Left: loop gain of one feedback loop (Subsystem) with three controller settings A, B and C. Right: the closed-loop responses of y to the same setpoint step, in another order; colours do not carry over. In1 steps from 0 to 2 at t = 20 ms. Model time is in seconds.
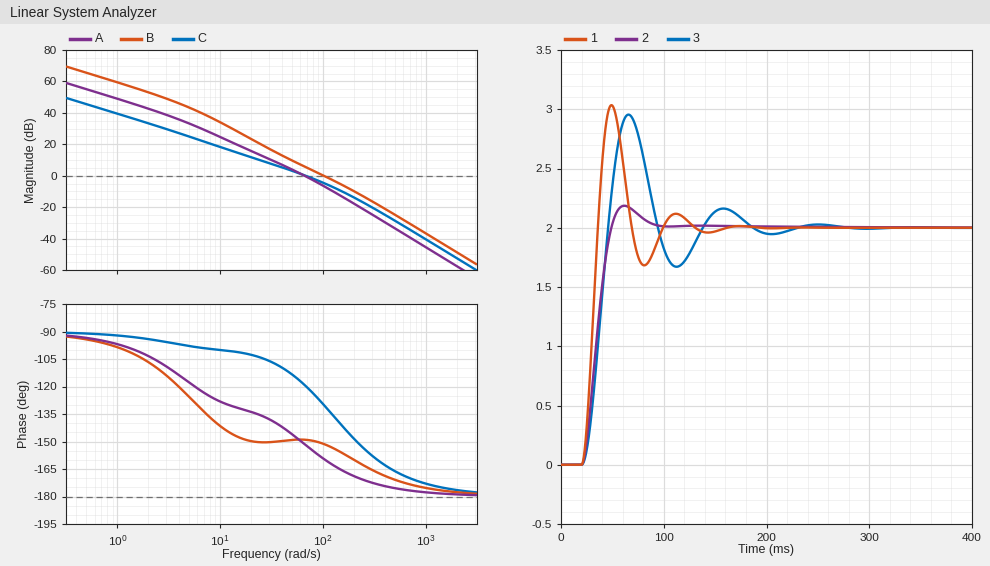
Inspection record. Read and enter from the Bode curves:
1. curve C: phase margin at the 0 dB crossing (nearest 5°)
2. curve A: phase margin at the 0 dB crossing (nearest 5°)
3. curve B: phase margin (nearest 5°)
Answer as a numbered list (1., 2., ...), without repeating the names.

1. 60°
2. 30°
3. 30°
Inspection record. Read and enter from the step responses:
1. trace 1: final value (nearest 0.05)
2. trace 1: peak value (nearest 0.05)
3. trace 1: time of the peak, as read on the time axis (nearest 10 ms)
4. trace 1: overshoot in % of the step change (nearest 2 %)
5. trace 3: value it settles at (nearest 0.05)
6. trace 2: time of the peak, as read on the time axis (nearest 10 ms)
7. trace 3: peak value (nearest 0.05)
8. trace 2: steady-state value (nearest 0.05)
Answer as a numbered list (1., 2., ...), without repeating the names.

1. 2.00
2. 3.05
3. 50 ms
4. 52 %
5. 2.00
6. 60 ms
7. 2.95
8. 2.00
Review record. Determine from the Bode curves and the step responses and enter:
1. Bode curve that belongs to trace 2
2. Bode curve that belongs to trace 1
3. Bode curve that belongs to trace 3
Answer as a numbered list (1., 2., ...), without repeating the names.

1. C
2. B
3. A
